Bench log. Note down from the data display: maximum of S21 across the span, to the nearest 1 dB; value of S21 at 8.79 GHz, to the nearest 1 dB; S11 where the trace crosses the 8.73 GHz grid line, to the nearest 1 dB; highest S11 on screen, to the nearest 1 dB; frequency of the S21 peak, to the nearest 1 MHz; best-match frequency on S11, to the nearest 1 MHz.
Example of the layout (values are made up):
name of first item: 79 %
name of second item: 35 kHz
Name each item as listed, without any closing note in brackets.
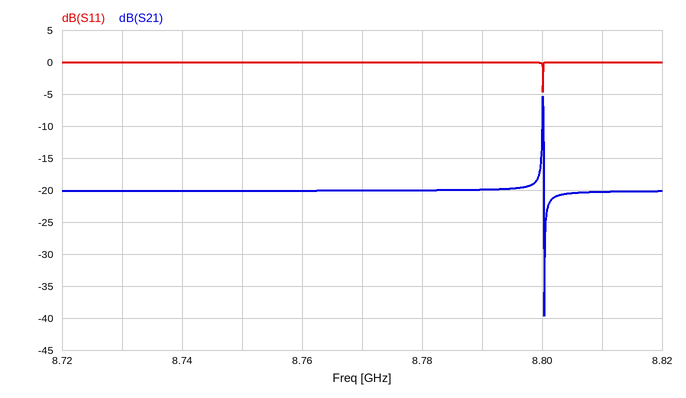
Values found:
maximum of S21 across the span, to the nearest 1 dB: -5 dB
value of S21 at 8.79 GHz, to the nearest 1 dB: -20 dB
S11 where the trace crosses the 8.73 GHz grid line, to the nearest 1 dB: 0 dB
highest S11 on screen, to the nearest 1 dB: 0 dB
frequency of the S21 peak, to the nearest 1 MHz: 8.800 GHz
best-match frequency on S11, to the nearest 1 MHz: 8.800 GHz
